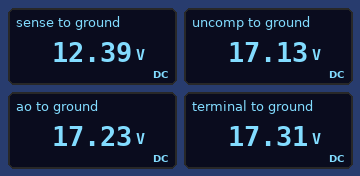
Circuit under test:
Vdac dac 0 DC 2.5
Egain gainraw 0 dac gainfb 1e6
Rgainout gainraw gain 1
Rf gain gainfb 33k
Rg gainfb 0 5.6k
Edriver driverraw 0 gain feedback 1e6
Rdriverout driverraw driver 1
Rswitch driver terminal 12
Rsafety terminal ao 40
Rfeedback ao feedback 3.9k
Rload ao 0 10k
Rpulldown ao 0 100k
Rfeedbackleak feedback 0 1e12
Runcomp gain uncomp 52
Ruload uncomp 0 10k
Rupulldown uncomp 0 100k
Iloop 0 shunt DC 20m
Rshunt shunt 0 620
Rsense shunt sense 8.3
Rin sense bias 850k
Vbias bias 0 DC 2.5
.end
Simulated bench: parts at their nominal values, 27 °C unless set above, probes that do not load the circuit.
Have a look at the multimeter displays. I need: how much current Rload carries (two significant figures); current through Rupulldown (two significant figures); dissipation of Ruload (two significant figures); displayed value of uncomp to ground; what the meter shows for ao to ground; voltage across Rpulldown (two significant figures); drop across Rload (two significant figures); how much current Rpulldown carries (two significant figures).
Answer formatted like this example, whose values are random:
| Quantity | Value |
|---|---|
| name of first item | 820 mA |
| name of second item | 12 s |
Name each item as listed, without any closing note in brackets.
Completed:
| Quantity | Value |
|---|---|
| how much current Rload carries | 1.7 mA |
| current through Rupulldown | 170 µA |
| dissipation of Ruload | 29 mW |
| displayed value of uncomp to ground | 17.13 V |
| what the meter shows for ao to ground | 17.23 V |
| voltage across Rpulldown | 17 V |
| drop across Rload | 17 V |
| how much current Rpulldown carries | 170 µA |
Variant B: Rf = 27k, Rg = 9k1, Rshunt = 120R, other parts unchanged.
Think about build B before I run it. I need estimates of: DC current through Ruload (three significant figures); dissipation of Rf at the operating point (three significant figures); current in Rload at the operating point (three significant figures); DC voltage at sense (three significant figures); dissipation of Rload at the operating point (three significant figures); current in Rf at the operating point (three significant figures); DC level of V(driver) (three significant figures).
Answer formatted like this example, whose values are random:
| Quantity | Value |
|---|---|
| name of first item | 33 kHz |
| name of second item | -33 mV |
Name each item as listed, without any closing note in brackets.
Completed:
| Quantity | Value |
|---|---|
| DC current through Ruload | 986 µA |
| dissipation of Rf at the operating point | 2.04 mW |
| current in Rload at the operating point | 992 µA |
| DC voltage at sense | 2.40 V |
| dissipation of Rload at the operating point | 9.84 mW |
| current in Rf at the operating point | 275 µA |
| DC level of V(driver) | 9.97 V |
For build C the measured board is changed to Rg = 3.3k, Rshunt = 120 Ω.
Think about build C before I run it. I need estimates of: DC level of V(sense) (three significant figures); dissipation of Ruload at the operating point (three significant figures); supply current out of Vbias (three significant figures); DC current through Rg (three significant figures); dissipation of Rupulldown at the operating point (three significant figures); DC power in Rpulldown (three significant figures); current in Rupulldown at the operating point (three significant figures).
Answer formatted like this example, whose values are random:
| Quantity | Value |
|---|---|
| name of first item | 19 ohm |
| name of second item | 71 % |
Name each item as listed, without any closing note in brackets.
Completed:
| Quantity | Value |
|---|---|
| DC level of V(sense) | 2.40 V |
| dissipation of Ruload at the operating point | 74.8 mW |
| supply current out of Vbias | 118 nA |
| DC current through Rg | 758 µA |
| dissipation of Rupulldown at the operating point | 7.48 mW |
| DC power in Rpulldown | 7.56 mW |
| current in Rupulldown at the operating point | 273 µA |
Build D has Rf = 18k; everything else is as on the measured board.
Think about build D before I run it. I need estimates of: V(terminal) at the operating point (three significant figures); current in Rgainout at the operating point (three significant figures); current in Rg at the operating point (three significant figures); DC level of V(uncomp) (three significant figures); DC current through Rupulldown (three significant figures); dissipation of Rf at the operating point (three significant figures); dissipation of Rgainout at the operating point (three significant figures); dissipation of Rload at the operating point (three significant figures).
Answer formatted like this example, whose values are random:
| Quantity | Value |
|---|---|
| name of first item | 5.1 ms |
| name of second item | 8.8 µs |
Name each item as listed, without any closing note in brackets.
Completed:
| Quantity | Value |
|---|---|
| V(terminal) at the operating point | 10.6 V |
| current in Rgainout at the operating point | 1.60 mA |
| current in Rg at the operating point | 446 µA |
| DC level of V(uncomp) | 10.5 V |
| DC current through Rupulldown | 105 µA |
| dissipation of Rf at the operating point | 3.59 mW |
| dissipation of Rgainout at the operating point | 2.56 µW |
| dissipation of Rload at the operating point | 11.1 mW |
